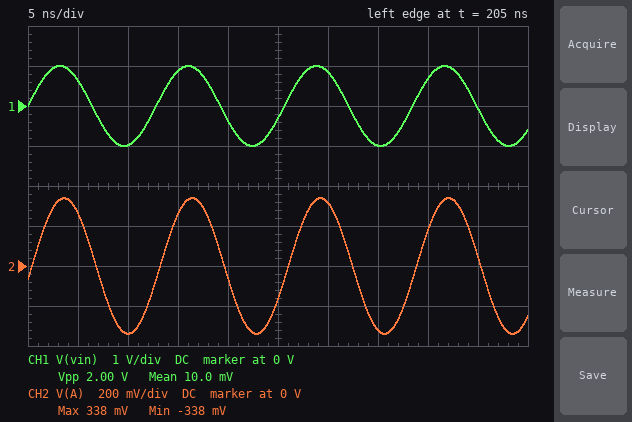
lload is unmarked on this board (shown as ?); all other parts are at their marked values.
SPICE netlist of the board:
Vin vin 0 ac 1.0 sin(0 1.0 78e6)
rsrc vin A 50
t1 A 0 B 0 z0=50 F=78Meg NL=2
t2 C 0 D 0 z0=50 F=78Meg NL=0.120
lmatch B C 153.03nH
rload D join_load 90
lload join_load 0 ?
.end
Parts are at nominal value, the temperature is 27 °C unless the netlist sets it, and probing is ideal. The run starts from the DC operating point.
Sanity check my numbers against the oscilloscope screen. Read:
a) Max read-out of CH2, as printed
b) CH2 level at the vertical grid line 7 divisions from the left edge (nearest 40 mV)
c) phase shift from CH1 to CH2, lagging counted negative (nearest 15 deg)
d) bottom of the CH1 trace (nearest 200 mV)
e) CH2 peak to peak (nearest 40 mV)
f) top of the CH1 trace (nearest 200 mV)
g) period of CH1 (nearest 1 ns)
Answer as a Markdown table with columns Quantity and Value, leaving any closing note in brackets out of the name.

| Quantity | Value |
|---|---|
| Max read-out of CH2, as printed | 338 mV |
| CH2 level at the vertical grid line 7 divisions from the left edge | -320 mV |
| phase shift from CH1 to CH2, lagging counted negative | -15 deg |
| bottom of the CH1 trace | -1.0 V |
| CH2 peak to peak | 680 mV |
| top of the CH1 trace | 1.0 V |
| period of CH1 | 13 ns |
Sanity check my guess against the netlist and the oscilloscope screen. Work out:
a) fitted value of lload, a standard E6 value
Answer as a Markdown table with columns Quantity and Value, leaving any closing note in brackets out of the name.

| Quantity | Value |
|---|---|
| fitted value of lload, a standard E6 value | 330 nH |
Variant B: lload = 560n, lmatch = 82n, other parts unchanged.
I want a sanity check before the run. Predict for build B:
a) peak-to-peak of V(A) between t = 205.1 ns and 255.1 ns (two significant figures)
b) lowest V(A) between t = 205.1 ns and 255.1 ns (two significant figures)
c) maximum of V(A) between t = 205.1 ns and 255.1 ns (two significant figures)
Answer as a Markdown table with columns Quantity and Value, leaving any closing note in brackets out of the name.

| Quantity | Value |
|---|---|
| peak-to-peak of V(A) between t = 205.1 ns and 255.1 ns | 1.0 V |
| lowest V(A) between t = 205.1 ns and 255.1 ns | -520 mV |
| maximum of V(A) between t = 205.1 ns and 255.1 ns | 520 mV |
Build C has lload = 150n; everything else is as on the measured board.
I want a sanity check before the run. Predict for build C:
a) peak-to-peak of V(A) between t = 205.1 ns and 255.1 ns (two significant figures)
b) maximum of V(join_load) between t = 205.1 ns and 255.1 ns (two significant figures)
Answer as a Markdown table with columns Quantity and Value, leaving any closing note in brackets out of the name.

| Quantity | Value |
|---|---|
| peak-to-peak of V(A) between t = 205.1 ns and 255.1 ns | 1.1 V |
| maximum of V(join_load) between t = 205.1 ns and 255.1 ns | 550 mV |
